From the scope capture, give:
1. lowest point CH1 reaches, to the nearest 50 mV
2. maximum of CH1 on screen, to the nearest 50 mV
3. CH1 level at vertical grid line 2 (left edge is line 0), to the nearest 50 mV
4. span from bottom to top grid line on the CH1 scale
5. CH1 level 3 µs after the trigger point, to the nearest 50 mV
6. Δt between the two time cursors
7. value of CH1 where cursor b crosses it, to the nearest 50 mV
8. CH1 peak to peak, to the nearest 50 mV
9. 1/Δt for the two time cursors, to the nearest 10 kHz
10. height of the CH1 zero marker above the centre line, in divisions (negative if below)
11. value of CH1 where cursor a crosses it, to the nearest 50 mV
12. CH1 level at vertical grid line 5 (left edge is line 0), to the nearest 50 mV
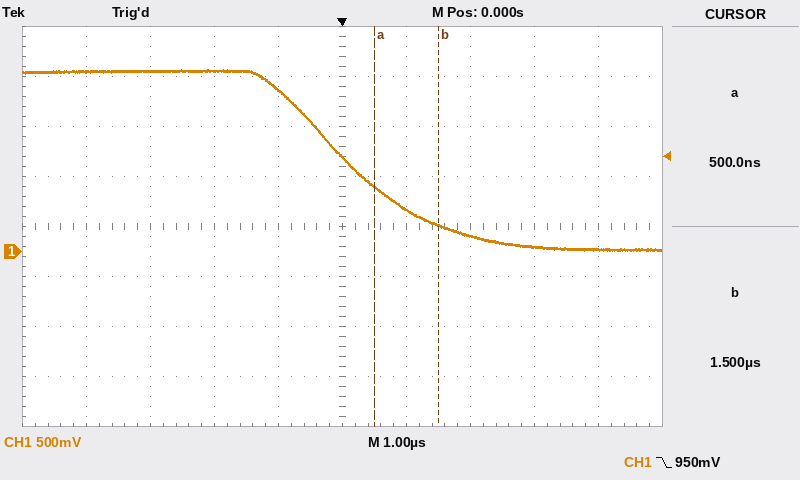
0 mV
1.80 V
1.80 V
4 V
50 mV
1.0 µs
250 mV
1.80 V
1.00 MHz
-0.5 div
650 mV
950 mV
